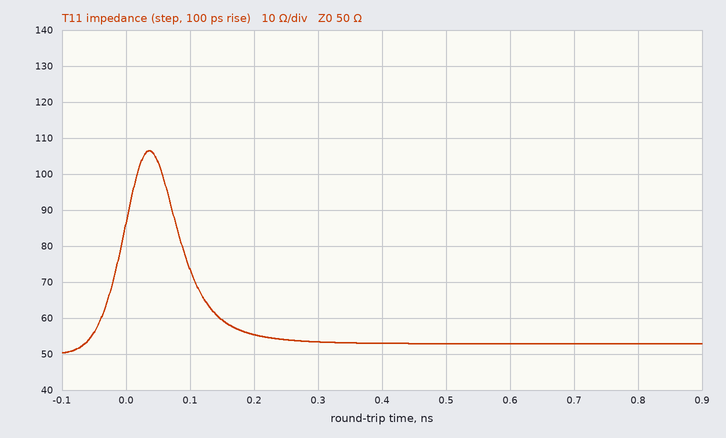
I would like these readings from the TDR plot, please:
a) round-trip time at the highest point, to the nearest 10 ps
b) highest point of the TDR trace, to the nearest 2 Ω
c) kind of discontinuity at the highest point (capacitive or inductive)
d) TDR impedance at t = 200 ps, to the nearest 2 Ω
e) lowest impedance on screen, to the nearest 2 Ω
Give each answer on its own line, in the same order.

40 ps
106 Ω
inductive
56 Ω
50 Ω
